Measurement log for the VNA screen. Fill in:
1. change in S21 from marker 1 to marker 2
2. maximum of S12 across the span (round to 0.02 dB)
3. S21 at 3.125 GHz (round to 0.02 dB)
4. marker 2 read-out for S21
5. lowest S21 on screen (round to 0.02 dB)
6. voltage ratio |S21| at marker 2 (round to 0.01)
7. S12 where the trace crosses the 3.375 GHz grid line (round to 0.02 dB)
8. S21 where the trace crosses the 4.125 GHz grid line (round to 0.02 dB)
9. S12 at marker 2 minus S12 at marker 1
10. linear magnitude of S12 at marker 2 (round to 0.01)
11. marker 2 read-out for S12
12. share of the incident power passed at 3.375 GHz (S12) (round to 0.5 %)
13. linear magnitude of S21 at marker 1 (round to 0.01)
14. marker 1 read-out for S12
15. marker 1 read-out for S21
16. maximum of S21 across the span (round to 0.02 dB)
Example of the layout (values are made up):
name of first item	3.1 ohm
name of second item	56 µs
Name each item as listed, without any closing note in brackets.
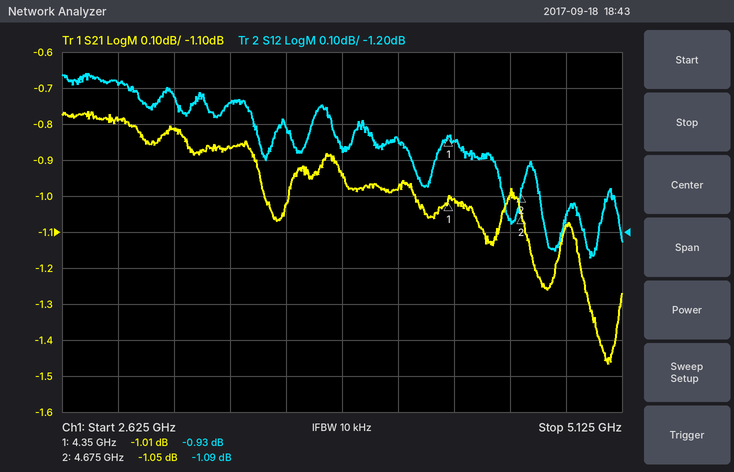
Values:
change in S21 from marker 1 to marker 2	-0.04 dB
maximum of S12 across the span	-0.76 dB
S21 at 3.125 GHz	-0.82 dB
marker 2 read-out for S21	-1.05 dB
lowest S21 on screen	-1.46 dB
voltage ratio |S21| at marker 2	0.89
S12 where the trace crosses the 3.375 GHz grid line	-0.84 dB
S21 where the trace crosses the 4.125 GHz grid line	-0.98 dB
S12 at marker 2 minus S12 at marker 1	-0.16 dB
linear magnitude of S12 at marker 2	0.88
marker 2 read-out for S12	-1.09 dB
share of the incident power passed at 3.375 GHz (S12)	82.5 %
linear magnitude of S21 at marker 1	0.89
marker 1 read-out for S12	-0.93 dB
marker 1 read-out for S21	-1.01 dB
maximum of S21 across the span	-0.76 dB
